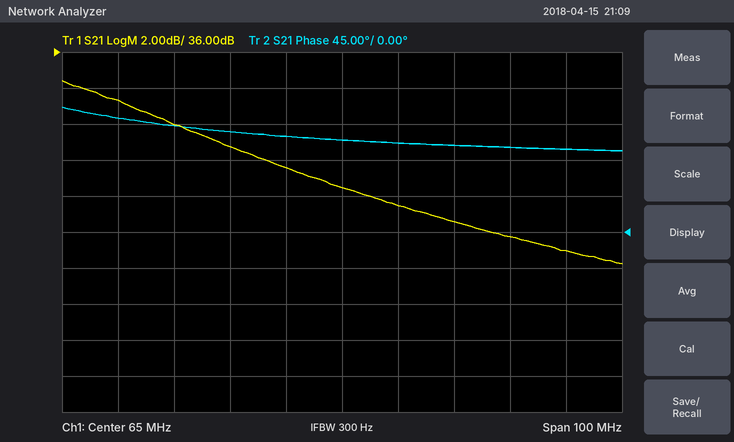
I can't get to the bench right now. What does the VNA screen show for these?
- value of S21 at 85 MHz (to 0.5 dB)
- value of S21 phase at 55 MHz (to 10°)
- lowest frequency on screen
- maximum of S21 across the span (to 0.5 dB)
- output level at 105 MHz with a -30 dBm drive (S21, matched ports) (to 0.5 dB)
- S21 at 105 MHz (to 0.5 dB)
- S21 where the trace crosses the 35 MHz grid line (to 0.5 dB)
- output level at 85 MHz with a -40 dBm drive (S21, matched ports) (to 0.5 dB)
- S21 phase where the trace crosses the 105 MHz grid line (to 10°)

26.5 dB
120°
15 MHz
34.5 dB
-5.0 dBm
25.0 dB
32.0 dB
-13.5 dBm
100°
